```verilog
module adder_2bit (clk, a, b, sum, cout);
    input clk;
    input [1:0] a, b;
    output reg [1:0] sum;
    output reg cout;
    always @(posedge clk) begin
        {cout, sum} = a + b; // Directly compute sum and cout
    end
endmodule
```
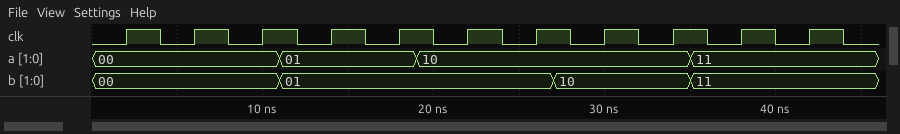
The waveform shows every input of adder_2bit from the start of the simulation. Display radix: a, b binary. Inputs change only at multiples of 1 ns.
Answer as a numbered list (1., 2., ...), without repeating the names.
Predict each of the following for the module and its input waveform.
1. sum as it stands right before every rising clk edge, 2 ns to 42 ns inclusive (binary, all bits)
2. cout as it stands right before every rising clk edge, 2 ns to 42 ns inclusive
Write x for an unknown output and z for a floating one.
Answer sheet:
1. x, 00, 00, 00, 10, 10, 11, 11, 00, 00, 10
2. x 0 0 0 0 0 0 0 1 1 1
